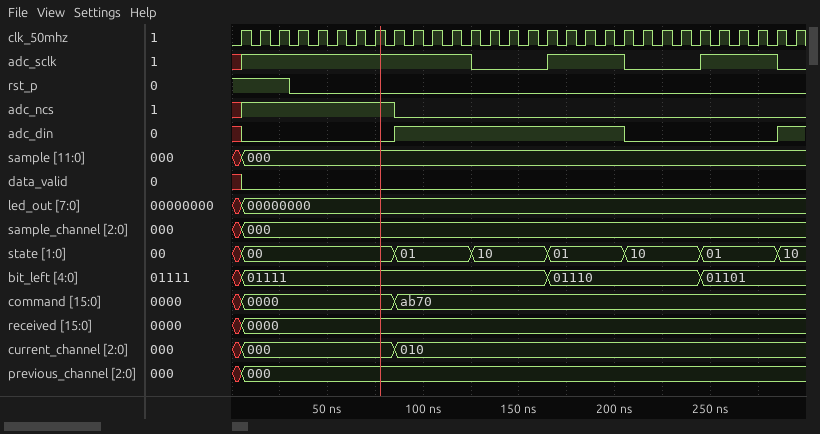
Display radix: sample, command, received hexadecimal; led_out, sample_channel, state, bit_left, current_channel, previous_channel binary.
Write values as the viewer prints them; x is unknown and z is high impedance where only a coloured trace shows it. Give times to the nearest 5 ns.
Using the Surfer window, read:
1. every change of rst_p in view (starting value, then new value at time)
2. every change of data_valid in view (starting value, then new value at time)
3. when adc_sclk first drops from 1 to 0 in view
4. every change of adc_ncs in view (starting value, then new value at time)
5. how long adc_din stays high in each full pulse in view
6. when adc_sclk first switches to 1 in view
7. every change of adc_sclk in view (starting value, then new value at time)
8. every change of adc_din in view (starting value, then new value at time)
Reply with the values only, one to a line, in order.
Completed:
1, 0 at 30 ns
x, 0 at 5 ns
125 ns
x, 1 at 5 ns, 0 at 85 ns
120 ns
5 ns
x, 1 at 5 ns, 0 at 125 ns, 1 at 165 ns, 0 at 205 ns, 1 at 245 ns, 0 at 285 ns
x, 0 at 5 ns, 1 at 85 ns, 0 at 205 ns, 1 at 285 ns
